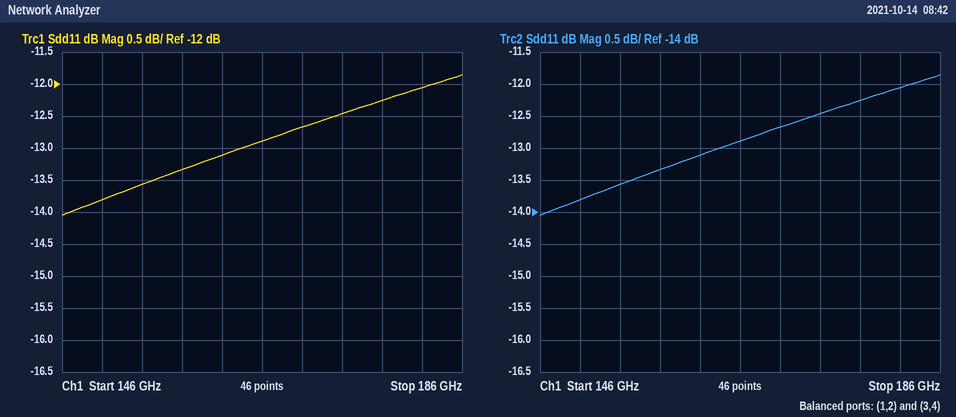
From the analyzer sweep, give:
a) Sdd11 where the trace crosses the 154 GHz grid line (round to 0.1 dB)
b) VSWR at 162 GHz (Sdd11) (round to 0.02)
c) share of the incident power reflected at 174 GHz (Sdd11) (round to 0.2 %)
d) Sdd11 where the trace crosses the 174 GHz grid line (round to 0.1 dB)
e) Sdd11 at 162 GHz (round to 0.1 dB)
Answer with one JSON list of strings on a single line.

["-13.6 dB", "1.56", "5.6 %", "-12.5 dB", "-13.1 dB"]
